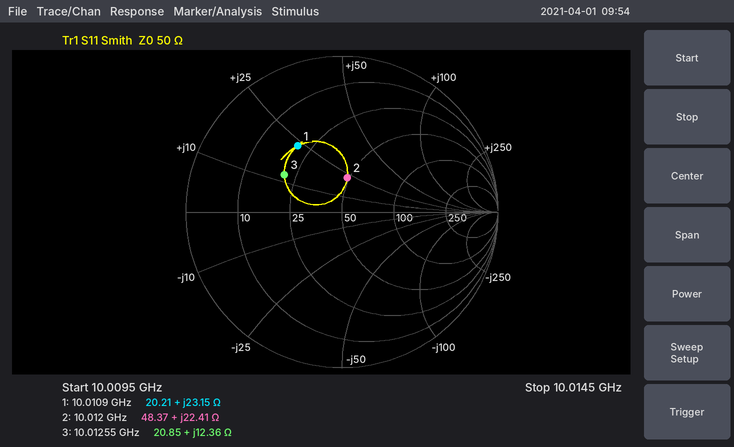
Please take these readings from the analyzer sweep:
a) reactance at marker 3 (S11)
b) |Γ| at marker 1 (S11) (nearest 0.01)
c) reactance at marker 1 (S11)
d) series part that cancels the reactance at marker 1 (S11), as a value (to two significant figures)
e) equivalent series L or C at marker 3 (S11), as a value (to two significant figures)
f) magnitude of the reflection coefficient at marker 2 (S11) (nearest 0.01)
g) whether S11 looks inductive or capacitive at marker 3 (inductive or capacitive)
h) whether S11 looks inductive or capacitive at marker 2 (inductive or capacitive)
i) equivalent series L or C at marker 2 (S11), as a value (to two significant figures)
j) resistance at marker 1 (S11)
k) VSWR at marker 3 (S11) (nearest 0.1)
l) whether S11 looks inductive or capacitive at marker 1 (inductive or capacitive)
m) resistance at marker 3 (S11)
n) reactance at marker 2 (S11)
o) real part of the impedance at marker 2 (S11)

+12.36 Ω
0.51
+23.15 Ω
690 fF
200 pH
0.22
inductive
inductive
360 pH
20.21 Ω
2.6
inductive
20.85 Ω
+22.41 Ω
48.37 Ω
